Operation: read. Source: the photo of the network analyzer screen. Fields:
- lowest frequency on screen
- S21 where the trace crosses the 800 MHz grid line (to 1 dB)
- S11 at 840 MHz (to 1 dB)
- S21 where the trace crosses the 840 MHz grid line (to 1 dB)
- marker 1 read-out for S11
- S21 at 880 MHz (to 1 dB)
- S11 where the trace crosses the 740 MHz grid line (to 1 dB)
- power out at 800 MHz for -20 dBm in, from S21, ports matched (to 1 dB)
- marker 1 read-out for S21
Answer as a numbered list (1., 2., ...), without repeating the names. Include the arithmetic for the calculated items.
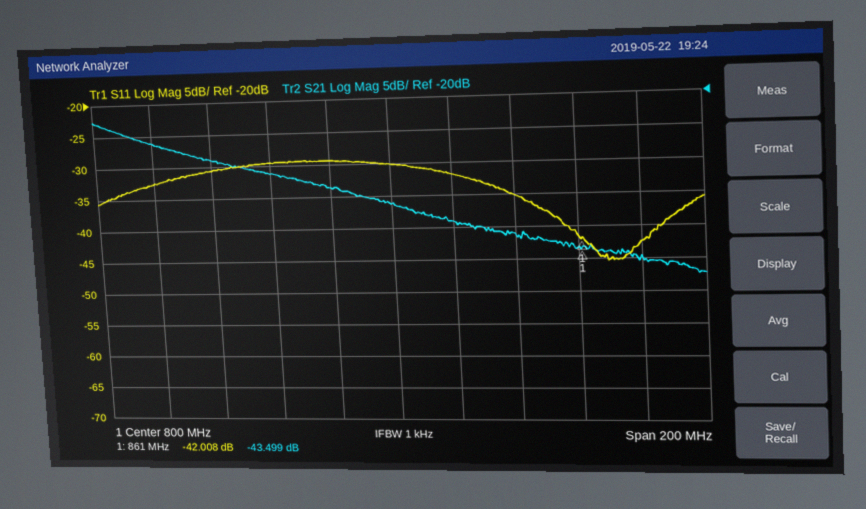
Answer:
1. 700 MHz
2. -36 dB
3. -35 dB
4. -41 dB
5. -42.008 dB
6. -45 dB
7. -31 dB
8. -20 dBm + (-36 dB) = -56 dBm
9. -43.499 dB
